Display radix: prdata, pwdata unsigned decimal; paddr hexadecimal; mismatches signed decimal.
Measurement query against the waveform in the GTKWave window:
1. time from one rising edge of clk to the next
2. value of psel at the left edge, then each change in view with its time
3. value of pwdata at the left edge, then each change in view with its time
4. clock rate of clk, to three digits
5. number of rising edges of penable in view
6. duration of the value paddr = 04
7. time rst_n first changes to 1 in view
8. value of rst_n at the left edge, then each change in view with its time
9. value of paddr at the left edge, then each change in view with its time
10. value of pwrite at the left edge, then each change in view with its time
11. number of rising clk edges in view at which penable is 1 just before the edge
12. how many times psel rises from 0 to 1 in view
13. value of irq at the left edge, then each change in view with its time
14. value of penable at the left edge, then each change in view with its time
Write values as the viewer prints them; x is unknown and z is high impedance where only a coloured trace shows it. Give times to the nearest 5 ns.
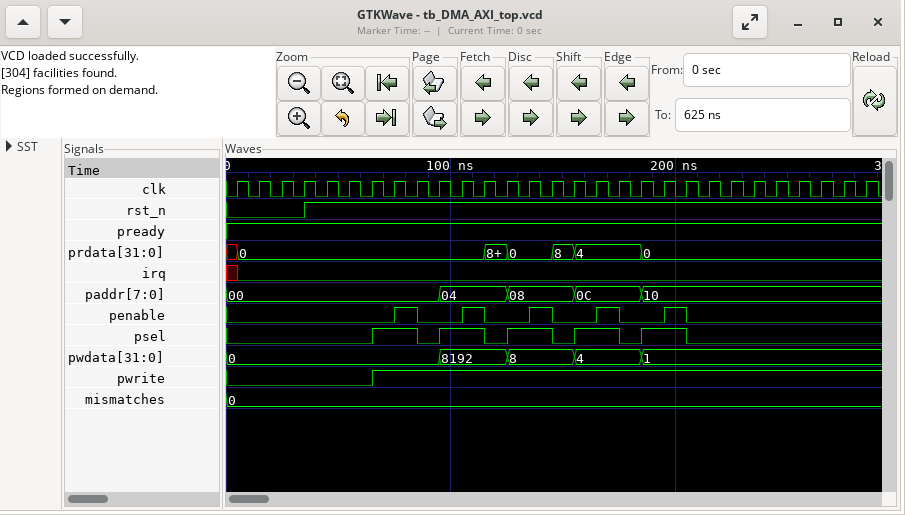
10 ns
0, 1 at 65 ns, 0 at 85 ns, 1 at 95 ns, 0 at 115 ns, 1 at 125 ns, 0 at 145 ns, 1 at 155 ns, 0 at 175 ns, 1 at 185 ns, 0 at 205 ns
0, 8192 at 95 ns, 8 at 125 ns, 4 at 155 ns, 1 at 185 ns
100 MHz
5
30 ns
35 ns
0, 1 at 35 ns
00, 04 at 95 ns, 08 at 125 ns, 0C at 155 ns, 10 at 185 ns
0, 1 at 65 ns
5
5
x, 0 at 5 ns
0, 1 at 75 ns, 0 at 85 ns, 1 at 105 ns, 0 at 115 ns, 1 at 135 ns, 0 at 145 ns, 1 at 165 ns, 0 at 175 ns, 1 at 195 ns, 0 at 205 ns
